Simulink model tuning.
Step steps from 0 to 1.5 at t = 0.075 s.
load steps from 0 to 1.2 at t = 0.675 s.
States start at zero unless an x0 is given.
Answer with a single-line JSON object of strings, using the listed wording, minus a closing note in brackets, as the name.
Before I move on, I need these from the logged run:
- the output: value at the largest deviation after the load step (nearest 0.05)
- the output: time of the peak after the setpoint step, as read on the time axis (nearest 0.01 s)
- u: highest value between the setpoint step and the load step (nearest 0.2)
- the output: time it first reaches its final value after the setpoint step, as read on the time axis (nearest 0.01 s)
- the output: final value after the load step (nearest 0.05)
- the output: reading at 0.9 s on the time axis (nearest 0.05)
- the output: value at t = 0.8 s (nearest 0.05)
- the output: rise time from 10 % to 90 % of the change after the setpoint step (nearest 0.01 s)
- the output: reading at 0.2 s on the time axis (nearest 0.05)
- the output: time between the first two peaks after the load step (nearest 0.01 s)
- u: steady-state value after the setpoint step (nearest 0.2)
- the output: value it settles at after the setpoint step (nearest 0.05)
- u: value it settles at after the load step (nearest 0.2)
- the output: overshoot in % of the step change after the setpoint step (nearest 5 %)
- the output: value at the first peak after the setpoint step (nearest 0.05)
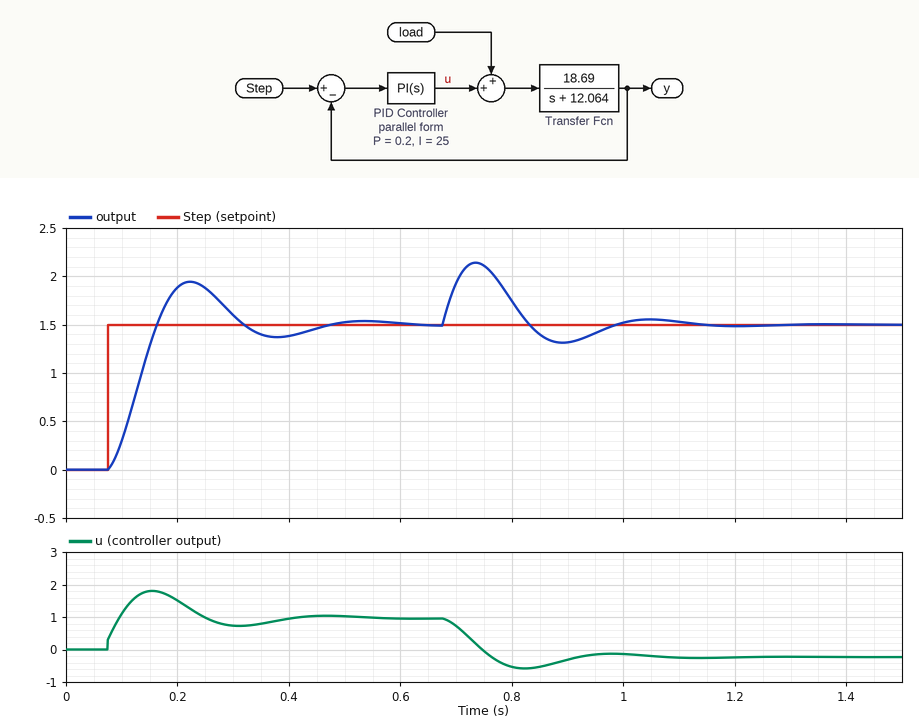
{"the output: value at the largest deviation after the load step": "2.15", "the output: time of the peak after the setpoint step, as read on the time axis": "0.22 s", "u: highest value between the setpoint step and the load step": "1.8", "the output: time it first reaches its final value after the setpoint step, as read on the time axis": "0.16 s", "the output: final value after the load step": "1.50", "the output: reading at 0.9 s on the time axis": "1.30", "the output: value at t = 0.8 s": "1.75", "the output: rise time from 10 % to 90 % of the change after the setpoint step": "0.06 s", "the output: reading at 0.2 s on the time axis": "1.90", "the output: time between the first two peaks after the load step": "0.31 s", "u: steady-state value after the setpoint step": "1.0", "the output: value it settles at after the setpoint step": "1.50", "u: value it settles at after the load step": "-0.2", "the output: overshoot in % of the step change after the setpoint step": "30 %", "the output: value at the first peak after the setpoint step": "1.95"}
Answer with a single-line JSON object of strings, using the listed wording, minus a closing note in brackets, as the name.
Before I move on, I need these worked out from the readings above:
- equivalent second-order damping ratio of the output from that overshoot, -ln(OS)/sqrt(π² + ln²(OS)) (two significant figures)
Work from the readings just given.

{"equivalent second-order damping ratio of the output from that overshoot, -ln(OS)/sqrt(π² + ln²(OS))": "0.36"}
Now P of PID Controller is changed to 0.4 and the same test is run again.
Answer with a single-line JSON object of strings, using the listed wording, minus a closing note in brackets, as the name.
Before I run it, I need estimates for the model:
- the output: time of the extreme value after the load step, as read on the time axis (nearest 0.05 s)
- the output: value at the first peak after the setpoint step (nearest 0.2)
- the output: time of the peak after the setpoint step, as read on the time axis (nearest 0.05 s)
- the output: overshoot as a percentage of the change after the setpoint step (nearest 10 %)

{"the output: time of the extreme value after the load step, as read on the time axis": "0.75 s", "the output: value at the first peak after the setpoint step": "1.8", "the output: time of the peak after the setpoint step, as read on the time axis": "0.20 s", "the output: overshoot as a percentage of the change after the setpoint step": "20 %"}
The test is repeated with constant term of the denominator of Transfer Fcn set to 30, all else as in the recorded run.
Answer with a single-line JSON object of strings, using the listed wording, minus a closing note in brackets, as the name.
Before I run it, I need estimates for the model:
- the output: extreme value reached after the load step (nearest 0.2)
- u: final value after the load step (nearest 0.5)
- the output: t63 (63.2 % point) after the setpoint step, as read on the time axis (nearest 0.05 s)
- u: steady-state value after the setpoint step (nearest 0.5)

{"the output: extreme value reached after the load step": "2.0", "u: final value after the load step": "1.0", "the output: t63 (63.2 % point) after the setpoint step, as read on the time axis": "0.15 s", "u: steady-state value after the setpoint step": "2.5"}
